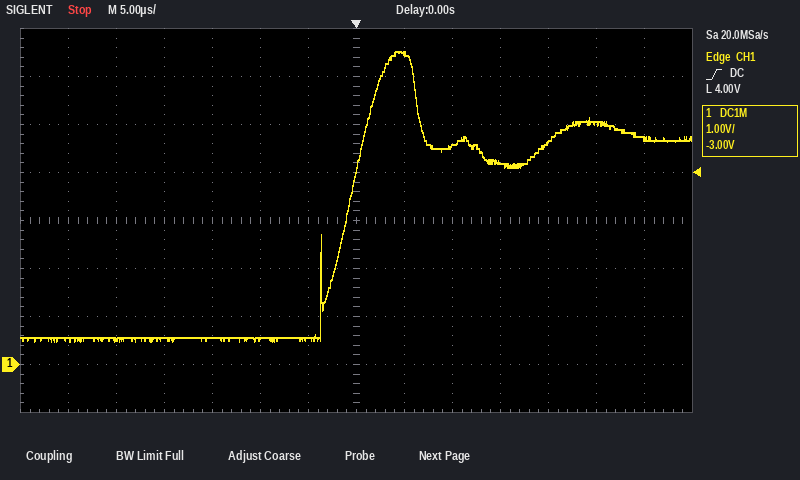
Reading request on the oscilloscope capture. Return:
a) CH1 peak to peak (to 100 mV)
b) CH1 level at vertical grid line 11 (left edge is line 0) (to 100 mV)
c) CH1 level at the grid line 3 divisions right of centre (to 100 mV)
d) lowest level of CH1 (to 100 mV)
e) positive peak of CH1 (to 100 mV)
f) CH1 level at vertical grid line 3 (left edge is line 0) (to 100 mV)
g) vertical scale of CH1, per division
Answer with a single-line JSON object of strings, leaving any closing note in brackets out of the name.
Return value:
{"CH1 peak to peak": "6.0 V", "CH1 level at vertical grid line 11 (left edge is line 0)": "4.6 V", "CH1 level at the grid line 3 divisions right of centre": "4.2 V", "lowest level of CH1": "500 mV", "positive peak of CH1": "6.5 V", "CH1 level at vertical grid line 3 (left edge is line 0)": "600 mV", "vertical scale of CH1, per division": "1 V"}
